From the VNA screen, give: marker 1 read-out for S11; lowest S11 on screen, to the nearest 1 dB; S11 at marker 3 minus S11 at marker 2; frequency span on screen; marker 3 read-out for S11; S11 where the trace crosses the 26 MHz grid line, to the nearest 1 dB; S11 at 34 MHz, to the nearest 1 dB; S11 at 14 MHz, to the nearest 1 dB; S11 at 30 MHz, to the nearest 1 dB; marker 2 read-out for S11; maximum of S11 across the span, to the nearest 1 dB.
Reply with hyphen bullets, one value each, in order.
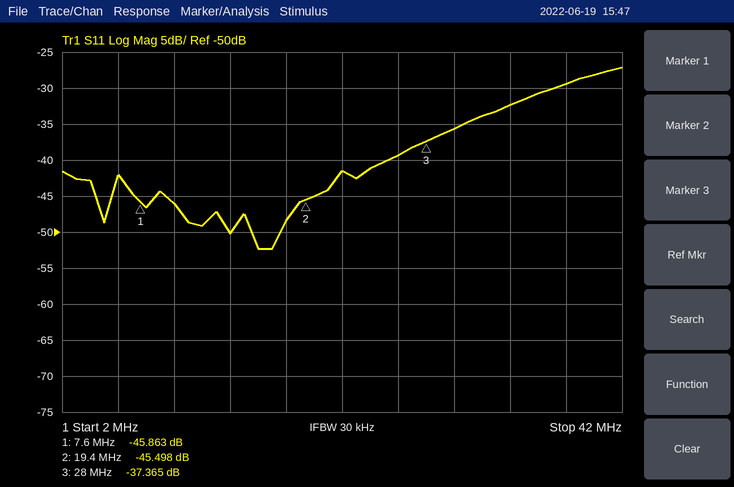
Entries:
- -45.863 dB
- -52 dB
- 8.133 dB
- 40 MHz
- -37.365 dB
- -39 dB
- -32 dB
- -50 dB
- -36 dB
- -45.498 dB
- -27 dB
